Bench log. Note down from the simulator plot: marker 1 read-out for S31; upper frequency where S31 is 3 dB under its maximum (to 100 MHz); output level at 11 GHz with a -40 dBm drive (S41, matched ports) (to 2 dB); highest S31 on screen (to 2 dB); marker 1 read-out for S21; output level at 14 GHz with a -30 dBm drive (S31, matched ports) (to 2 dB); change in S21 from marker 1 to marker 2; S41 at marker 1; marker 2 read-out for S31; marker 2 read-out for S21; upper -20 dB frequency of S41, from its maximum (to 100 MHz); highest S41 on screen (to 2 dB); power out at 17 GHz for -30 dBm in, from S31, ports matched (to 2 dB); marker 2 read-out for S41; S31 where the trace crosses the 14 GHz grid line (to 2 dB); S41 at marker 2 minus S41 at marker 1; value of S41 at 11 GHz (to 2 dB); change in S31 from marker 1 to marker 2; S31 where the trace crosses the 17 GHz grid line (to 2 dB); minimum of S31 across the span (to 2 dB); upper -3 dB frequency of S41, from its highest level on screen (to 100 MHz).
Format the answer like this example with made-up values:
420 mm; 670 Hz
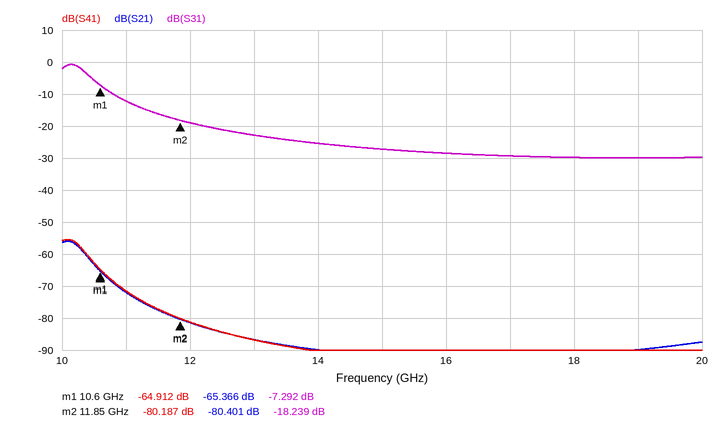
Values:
-7.292 dB; 10.4 GHz; -112 dBm; 0 dB; -65.366 dB; -56 dBm; -15.035 dB; -64.912 dB; -18.239 dB; -80.401 dB; 11.3 GHz; -56 dB; -60 dBm; -80.187 dB; -26 dB; -15.275 dB; -72 dB; -10.947 dB; -30 dB; -30 dB; 10.3 GHz
